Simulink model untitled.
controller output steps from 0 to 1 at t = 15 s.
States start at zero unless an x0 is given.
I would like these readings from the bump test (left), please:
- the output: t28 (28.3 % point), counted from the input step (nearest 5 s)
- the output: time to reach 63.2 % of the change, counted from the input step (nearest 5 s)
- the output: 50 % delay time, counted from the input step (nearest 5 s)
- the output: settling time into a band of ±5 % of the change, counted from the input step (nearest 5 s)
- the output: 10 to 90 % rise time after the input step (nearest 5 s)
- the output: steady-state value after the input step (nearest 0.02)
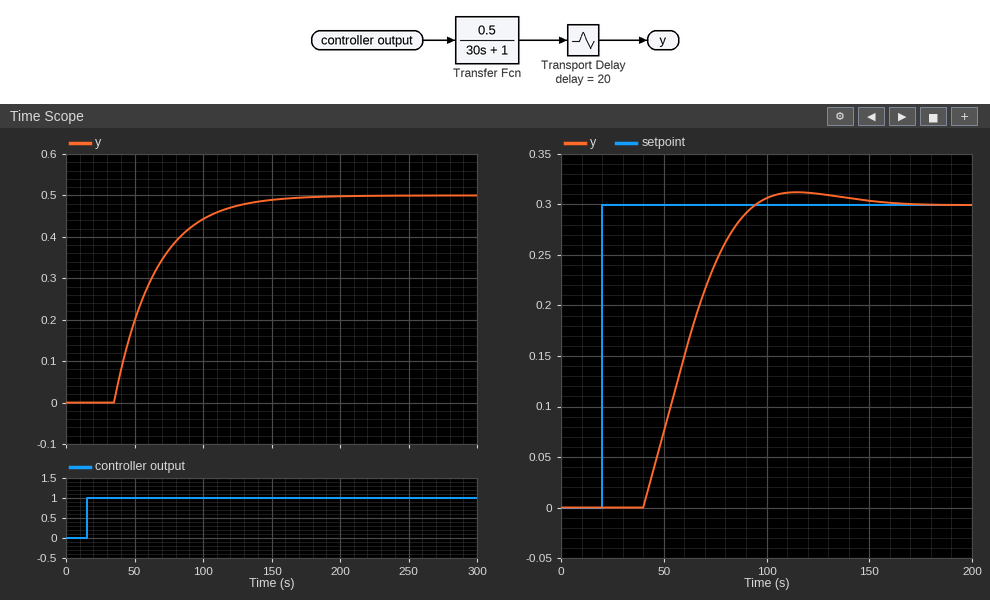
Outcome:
30 s
50 s
40 s
110 s
65 s
0.50
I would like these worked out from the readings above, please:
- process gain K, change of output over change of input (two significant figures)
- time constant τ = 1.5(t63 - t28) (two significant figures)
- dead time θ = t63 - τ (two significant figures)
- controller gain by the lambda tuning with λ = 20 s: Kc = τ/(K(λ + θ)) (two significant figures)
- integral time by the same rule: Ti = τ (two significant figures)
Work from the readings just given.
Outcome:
0.50
30 s
20 s
1.5
30 s
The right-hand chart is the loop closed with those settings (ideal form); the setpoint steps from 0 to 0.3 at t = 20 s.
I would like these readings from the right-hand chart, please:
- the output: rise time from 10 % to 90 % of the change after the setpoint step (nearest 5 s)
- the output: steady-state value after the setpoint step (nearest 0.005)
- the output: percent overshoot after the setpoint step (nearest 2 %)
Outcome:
40 s
0.300
4 %
